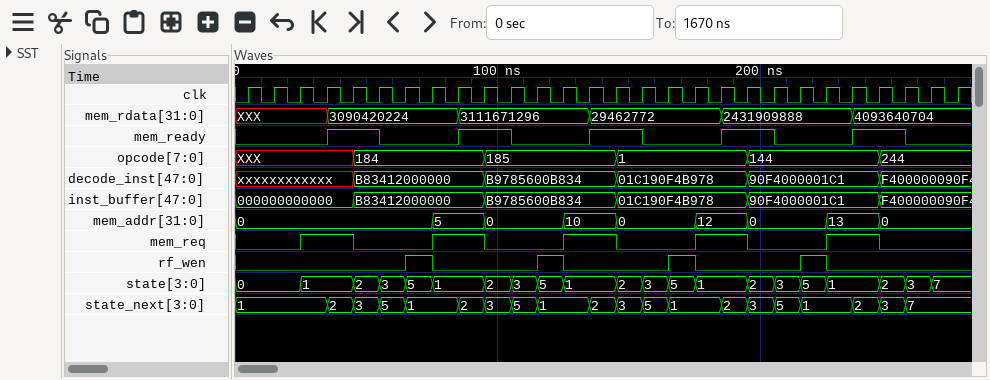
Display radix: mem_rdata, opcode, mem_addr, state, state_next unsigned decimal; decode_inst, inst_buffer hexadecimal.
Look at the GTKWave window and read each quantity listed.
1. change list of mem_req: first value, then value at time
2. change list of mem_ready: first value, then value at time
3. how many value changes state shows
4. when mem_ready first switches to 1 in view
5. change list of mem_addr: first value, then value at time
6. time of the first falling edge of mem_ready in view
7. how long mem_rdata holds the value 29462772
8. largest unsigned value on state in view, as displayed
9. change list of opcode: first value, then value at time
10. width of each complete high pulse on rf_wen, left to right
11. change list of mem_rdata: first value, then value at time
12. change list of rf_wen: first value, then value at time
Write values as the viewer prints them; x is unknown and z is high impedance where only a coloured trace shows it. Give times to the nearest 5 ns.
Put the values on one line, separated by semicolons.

0, 1 at 25 ns, 0 at 45 ns, 1 at 75 ns, 0 at 95 ns, 1 at 125 ns, 0 at 145 ns, 1 at 175 ns, 0 at 195 ns, 1 at 225 ns, 0 at 245 ns; 0, 1 at 35 ns, 0 at 55 ns, 1 at 85 ns, 0 at 105 ns, 1 at 135 ns, 0 at 155 ns, 1 at 185 ns, 0 at 205 ns, 1 at 235 ns, 0 at 255 ns; 20; 35 ns; 0, 5 at 75 ns, 0 at 95 ns, 10 at 125 ns, 0 at 145 ns, 12 at 175 ns, 0 at 195 ns, 13 at 225 ns, 0 at 245 ns; 55 ns; 50 ns; 7; XXX, 184 at 45 ns, 185 at 95 ns, 1 at 145 ns, 144 at 195 ns, 244 at 245 ns; 10 ns, 10 ns, 10 ns, 10 ns; XXX, 3090420224 at 35 ns, 3111671296 at 85 ns, 29462772 at 135 ns, 2431909888 at 185 ns, 4093640704 at 235 ns; 0, 1 at 65 ns, 0 at 75 ns, 1 at 115 ns, 0 at 125 ns, 1 at 165 ns, 0 at 175 ns, 1 at 215 ns, 0 at 225 ns
